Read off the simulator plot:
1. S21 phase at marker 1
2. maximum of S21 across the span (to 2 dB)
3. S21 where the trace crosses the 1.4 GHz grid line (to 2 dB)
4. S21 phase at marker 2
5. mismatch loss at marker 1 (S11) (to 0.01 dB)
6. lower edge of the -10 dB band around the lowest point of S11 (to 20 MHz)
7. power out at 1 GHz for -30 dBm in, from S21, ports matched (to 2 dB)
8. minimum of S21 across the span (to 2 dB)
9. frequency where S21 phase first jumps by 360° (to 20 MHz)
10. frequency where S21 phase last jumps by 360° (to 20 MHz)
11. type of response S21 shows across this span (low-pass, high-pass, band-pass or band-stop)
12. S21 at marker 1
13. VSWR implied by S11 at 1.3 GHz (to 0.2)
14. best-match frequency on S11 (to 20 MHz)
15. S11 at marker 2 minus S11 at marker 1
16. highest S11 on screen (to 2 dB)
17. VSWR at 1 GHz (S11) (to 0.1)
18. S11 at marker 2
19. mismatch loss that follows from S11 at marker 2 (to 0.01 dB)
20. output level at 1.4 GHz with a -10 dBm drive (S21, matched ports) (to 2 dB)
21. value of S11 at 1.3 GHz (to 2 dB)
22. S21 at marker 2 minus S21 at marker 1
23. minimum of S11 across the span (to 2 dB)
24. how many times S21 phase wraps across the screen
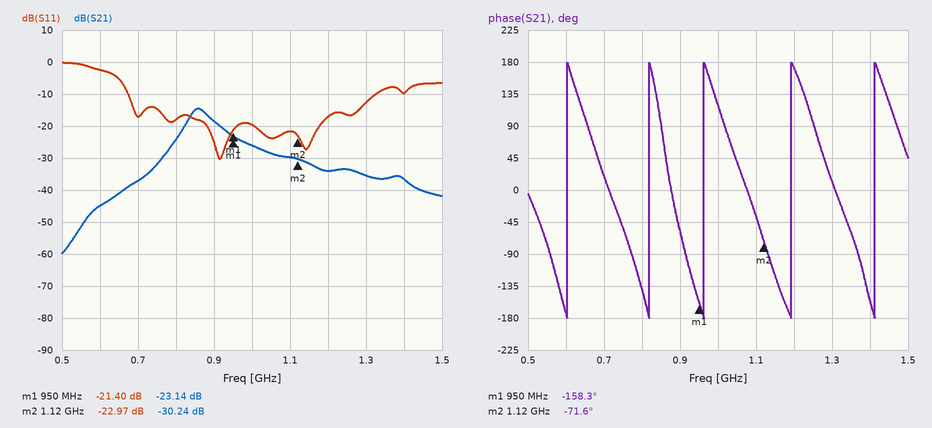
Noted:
-158.3°
-14 dB
-36 dB
-71.6°
0.03 dB
680 MHz
-56 dBm
-60 dB
600 MHz
1.42 GHz
band-pass
-23.14 dB
1.6
920 MHz
-1.57 dB
0 dB
1.2
-22.97 dB
0.02 dB
-46 dBm
-12 dB
-7.10 dB
-30 dB
5
